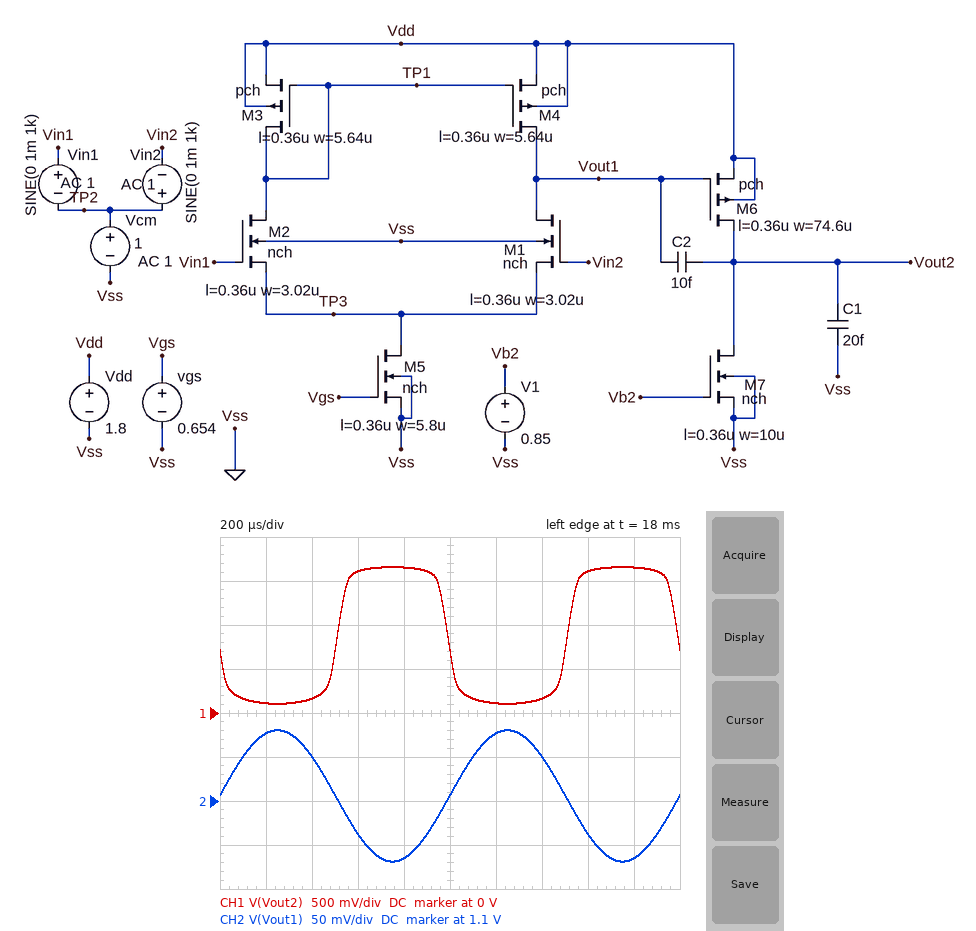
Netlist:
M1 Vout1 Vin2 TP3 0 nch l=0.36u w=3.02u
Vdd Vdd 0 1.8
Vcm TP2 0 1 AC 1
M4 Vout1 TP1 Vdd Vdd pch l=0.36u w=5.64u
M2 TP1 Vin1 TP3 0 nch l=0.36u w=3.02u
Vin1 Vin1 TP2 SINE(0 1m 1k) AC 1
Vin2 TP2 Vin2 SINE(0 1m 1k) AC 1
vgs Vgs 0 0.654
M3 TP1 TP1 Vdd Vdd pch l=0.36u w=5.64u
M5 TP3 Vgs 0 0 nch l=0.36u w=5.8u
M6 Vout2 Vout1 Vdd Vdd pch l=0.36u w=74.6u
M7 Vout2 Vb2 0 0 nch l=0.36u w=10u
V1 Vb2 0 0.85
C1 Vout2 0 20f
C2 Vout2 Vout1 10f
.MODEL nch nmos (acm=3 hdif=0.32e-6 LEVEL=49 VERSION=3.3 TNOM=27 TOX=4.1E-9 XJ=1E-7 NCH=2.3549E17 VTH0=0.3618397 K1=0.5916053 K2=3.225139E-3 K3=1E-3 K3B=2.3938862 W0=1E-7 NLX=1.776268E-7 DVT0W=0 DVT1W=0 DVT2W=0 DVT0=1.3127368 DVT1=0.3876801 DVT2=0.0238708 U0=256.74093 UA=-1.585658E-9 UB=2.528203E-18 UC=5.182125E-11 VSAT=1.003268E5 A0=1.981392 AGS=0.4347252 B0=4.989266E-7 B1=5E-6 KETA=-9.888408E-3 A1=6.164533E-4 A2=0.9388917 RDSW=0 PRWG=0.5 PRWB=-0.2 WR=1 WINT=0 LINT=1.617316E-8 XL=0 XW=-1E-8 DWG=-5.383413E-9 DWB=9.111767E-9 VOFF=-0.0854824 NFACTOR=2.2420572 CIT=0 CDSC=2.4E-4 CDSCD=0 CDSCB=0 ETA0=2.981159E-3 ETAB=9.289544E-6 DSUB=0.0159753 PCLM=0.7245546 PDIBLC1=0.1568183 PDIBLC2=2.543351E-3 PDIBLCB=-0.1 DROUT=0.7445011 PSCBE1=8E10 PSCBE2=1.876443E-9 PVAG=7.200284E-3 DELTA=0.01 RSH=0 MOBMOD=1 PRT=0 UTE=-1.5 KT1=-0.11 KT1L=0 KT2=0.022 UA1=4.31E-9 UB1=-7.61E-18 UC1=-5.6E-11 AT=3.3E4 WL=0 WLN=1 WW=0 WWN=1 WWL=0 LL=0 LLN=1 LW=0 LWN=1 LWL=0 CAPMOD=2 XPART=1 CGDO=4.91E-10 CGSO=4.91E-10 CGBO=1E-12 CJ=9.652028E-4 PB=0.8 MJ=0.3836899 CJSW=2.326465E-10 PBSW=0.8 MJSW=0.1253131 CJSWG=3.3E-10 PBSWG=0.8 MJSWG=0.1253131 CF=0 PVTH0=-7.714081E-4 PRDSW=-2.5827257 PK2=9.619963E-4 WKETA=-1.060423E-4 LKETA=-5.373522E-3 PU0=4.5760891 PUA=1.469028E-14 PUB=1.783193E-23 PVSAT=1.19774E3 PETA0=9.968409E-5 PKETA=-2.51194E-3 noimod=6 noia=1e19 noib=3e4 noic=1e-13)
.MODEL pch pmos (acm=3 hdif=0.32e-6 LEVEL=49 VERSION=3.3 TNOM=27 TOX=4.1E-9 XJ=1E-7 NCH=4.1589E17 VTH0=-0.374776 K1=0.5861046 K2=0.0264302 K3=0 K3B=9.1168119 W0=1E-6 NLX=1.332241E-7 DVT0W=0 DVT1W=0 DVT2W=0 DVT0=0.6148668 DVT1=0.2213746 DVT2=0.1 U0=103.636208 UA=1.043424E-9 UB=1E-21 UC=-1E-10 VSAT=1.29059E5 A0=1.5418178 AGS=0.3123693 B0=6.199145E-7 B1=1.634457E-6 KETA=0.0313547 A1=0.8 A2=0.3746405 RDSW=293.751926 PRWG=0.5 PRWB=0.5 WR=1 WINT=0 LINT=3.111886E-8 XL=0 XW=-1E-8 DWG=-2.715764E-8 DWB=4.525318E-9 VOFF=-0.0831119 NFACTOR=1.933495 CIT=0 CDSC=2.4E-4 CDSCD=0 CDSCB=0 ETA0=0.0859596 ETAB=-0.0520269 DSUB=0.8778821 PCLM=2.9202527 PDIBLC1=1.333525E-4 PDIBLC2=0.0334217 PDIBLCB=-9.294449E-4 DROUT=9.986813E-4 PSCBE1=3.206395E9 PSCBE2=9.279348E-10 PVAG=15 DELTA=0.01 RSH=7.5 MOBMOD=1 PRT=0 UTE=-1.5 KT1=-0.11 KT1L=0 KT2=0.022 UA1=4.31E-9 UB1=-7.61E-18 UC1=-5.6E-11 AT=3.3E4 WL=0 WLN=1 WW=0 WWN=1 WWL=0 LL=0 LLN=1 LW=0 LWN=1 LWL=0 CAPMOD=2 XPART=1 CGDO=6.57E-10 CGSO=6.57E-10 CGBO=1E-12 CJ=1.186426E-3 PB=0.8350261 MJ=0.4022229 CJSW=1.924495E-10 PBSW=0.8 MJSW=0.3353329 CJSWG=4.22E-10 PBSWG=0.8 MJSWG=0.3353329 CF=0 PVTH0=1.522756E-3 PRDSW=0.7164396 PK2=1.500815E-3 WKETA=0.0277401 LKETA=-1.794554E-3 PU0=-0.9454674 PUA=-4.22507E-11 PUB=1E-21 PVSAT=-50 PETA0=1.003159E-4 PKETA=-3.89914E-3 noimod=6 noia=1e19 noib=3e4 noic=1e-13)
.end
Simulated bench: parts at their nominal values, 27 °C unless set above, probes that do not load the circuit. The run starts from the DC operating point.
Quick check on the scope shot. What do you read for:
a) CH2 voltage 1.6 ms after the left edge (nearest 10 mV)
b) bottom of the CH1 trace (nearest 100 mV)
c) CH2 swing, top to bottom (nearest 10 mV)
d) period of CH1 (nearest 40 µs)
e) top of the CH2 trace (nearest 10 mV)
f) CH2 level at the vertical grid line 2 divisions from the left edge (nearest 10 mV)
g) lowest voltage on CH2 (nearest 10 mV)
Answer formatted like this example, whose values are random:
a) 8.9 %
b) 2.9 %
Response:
a) 1.06 V
b) 100 mV
c) 150 mV
d) 1.00 ms
e) 1.18 V
f) 1.15 V
g) 1.03 V
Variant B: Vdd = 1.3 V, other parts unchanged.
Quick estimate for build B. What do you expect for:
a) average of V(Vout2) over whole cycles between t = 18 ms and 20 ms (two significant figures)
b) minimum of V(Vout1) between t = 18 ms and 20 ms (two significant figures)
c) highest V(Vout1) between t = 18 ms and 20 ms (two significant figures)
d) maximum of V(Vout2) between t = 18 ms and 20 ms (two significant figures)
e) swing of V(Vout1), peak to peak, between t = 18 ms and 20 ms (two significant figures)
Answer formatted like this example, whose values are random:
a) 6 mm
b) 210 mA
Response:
a) 600 mV
b) 560 mV
c) 660 mV
d) 1.1 V
e) 110 mV
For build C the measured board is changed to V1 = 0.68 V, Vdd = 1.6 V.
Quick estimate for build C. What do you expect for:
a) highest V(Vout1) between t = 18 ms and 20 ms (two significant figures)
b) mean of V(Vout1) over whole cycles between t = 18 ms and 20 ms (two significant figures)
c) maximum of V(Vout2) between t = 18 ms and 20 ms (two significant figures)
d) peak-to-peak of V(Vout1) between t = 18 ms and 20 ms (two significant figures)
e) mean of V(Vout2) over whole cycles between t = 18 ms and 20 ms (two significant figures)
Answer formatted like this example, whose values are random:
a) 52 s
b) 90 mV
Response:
a) 980 mV
b) 910 mV
c) 1.6 V
d) 140 mV
e) 1.5 V
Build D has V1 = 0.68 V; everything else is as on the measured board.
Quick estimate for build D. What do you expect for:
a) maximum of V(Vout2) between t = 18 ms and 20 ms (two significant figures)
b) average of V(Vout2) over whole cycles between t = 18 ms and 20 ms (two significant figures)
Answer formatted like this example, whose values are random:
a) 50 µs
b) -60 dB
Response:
a) 1.8 V
b) 1.7 V
